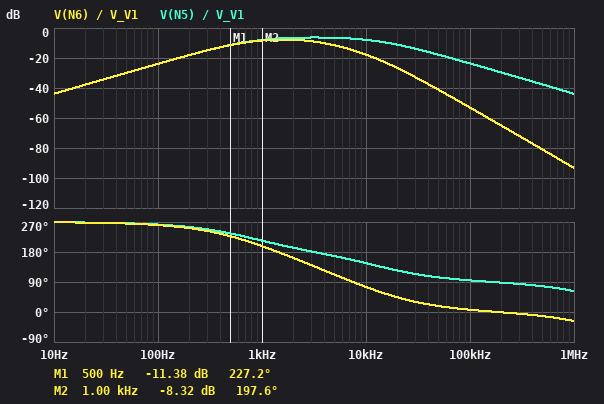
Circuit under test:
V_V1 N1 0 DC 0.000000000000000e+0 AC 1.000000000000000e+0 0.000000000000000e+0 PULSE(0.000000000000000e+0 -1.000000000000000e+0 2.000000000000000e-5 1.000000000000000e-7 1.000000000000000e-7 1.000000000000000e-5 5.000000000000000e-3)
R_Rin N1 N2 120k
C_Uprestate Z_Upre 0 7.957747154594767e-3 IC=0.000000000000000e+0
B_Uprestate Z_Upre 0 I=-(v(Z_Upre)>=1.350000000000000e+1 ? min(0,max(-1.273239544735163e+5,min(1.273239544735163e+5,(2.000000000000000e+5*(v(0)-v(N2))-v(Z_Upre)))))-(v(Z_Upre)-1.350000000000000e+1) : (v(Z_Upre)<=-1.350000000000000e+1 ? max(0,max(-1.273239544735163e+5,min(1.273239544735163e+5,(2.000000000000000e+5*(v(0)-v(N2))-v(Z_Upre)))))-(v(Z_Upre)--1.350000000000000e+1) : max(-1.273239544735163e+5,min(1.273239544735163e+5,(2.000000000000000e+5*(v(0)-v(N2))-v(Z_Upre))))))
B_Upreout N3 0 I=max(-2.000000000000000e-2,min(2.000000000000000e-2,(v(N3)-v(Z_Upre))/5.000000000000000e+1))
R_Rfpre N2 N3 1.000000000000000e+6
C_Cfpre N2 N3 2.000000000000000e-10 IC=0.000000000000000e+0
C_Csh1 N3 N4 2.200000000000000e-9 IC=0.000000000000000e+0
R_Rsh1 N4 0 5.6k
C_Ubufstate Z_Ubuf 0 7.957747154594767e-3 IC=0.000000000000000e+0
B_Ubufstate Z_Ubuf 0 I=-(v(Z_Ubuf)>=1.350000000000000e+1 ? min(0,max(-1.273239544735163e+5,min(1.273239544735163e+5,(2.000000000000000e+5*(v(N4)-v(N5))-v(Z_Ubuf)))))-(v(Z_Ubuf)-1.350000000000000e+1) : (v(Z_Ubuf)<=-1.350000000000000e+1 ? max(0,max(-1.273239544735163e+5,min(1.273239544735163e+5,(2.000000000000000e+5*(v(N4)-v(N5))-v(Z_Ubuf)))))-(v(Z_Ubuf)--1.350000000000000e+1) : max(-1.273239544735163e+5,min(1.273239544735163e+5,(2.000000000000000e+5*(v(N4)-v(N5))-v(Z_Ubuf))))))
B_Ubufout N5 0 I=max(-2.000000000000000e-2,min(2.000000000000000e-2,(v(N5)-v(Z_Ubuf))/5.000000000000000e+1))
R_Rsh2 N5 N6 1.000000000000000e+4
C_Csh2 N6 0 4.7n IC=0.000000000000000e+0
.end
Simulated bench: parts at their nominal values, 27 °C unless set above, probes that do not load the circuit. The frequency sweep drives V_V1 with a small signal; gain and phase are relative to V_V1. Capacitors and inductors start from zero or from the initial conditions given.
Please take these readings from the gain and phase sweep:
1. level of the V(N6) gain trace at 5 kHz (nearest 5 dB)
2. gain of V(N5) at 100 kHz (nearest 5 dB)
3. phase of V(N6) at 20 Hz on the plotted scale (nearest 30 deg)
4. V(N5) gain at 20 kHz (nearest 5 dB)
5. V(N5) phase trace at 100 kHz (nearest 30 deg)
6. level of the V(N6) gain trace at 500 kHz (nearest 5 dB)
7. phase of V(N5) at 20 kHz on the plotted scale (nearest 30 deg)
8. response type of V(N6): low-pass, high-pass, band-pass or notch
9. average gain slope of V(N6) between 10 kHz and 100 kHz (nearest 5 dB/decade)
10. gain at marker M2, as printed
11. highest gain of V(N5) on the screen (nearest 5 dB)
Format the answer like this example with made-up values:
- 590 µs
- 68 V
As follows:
- -10 dB
- -25 dB
- 270 deg
- -10 dB
- 90 deg
- -80 dB
- 120 deg
- band-pass
- -35 dB/decade
- -8.32 dB
- -5 dB
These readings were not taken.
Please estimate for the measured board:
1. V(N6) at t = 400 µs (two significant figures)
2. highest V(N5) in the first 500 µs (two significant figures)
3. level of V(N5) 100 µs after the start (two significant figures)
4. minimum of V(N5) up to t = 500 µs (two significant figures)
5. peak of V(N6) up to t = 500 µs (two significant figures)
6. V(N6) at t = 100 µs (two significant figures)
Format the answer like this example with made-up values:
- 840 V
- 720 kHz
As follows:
- -5.5 mV
- 280 mV
- -18 mV
- -18 mV
- 63 mV
- 15 mV
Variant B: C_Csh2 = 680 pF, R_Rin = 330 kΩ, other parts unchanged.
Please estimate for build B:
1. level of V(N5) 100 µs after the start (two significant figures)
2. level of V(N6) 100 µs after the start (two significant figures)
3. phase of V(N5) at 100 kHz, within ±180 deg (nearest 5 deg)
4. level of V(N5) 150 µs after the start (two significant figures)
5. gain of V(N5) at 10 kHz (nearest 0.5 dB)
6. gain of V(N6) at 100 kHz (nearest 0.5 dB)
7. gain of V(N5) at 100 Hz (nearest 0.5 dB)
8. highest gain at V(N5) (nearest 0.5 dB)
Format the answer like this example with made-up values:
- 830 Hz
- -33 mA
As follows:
- -6.5 mV
- -6.3 mV
- 95 deg
- -5.4 mV
- -16.5 dB
- -45.5 dB
- -32.5 dB
- -15.0 dB
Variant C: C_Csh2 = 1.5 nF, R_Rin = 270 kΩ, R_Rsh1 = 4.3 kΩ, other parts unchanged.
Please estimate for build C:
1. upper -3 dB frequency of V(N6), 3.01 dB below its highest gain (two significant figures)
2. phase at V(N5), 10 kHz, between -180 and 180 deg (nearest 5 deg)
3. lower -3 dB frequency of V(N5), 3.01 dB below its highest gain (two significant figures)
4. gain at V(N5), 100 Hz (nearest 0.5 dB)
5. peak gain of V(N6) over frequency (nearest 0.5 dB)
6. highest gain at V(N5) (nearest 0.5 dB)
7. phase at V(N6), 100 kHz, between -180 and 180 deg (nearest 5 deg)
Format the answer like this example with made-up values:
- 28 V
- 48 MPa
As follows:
- 9.4 kHz
- 155 deg
- 730 Hz
- -33.0 dB
- -16.0 dB
- -15.5 dB
- 15 deg
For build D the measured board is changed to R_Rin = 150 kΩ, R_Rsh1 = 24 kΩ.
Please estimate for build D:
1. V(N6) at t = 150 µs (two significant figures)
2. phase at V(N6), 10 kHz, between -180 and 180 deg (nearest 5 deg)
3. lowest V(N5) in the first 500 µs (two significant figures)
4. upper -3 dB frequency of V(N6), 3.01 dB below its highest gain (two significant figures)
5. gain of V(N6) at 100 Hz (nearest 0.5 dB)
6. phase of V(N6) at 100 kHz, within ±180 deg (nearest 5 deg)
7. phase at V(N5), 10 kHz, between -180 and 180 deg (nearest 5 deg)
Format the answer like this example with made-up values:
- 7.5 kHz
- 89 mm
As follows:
- 26 mV
- 40 deg
- -34 mV
- 3.0 kHz
- -13.0 dB
- 0 deg
- 110 deg
